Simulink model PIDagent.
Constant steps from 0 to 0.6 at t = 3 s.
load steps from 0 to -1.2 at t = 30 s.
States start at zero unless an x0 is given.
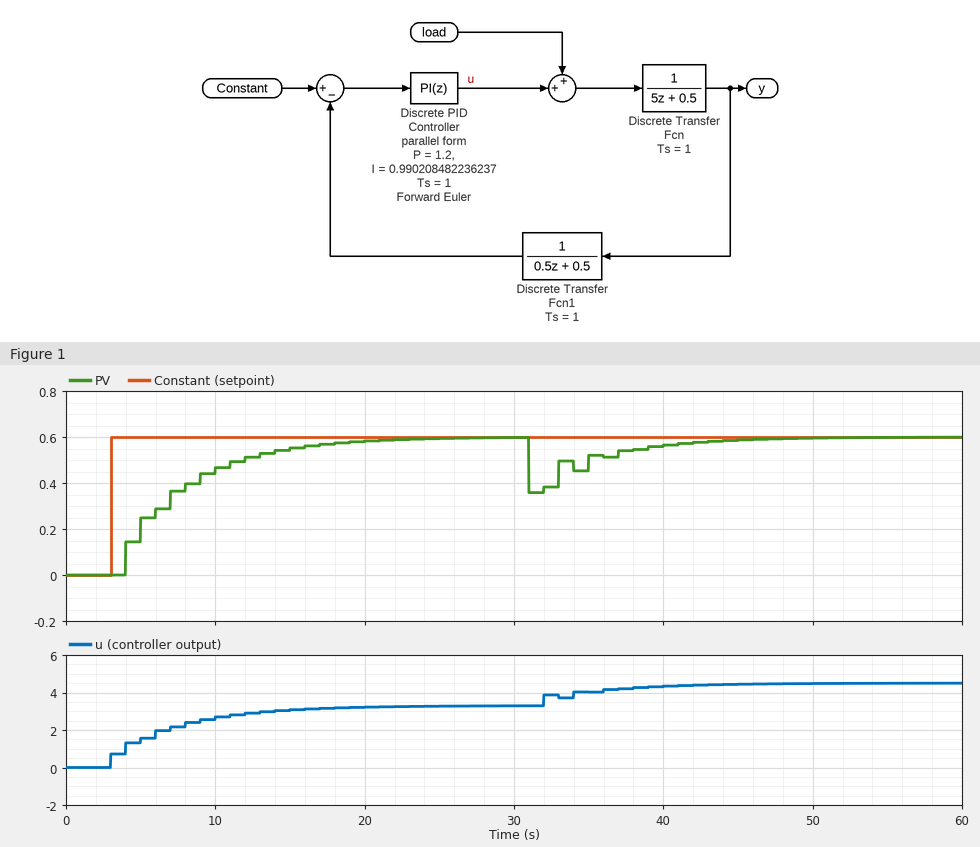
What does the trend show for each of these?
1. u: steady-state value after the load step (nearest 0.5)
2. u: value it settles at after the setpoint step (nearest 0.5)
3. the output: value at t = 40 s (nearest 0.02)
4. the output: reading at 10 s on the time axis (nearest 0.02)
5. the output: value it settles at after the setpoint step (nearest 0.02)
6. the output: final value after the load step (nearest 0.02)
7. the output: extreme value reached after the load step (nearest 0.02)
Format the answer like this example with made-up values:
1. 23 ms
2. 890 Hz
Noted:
1. 4.5
2. 3.5
3. 0.56
4. 0.46
5. 0.60
6. 0.60
7. 0.36
